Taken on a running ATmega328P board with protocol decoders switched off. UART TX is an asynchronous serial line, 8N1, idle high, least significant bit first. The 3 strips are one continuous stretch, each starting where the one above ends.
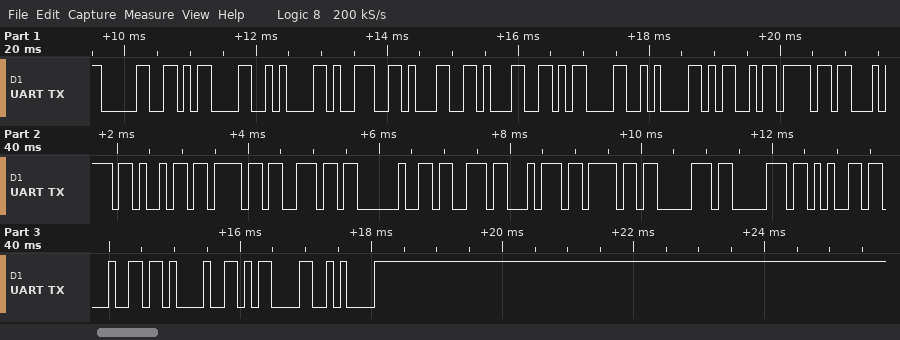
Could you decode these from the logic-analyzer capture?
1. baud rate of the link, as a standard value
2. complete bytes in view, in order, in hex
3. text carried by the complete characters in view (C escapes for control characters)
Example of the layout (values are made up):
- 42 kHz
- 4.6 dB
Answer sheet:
- 9600 baud
- 30 0D 0A 39 31 31 0D 0A 4D 6F 74 69 6F 6E 20 73 74 6F 70 70 65 64 21 0D 0A
- "0\r\n911\r\nMotion stopped!\r\n"
